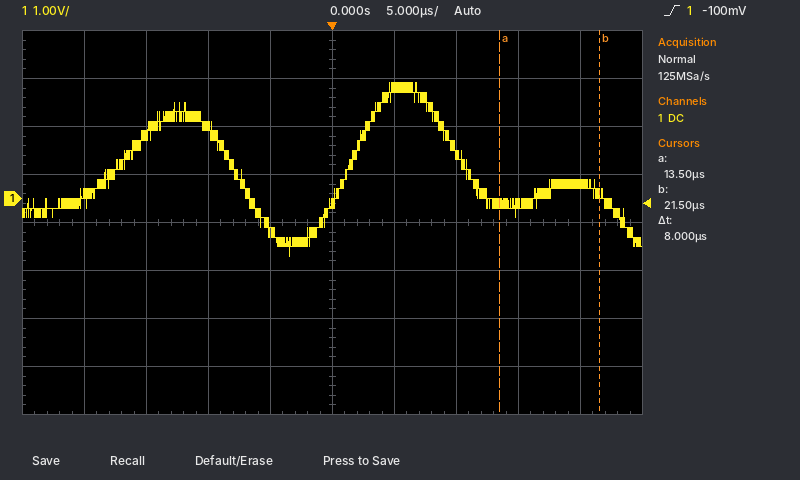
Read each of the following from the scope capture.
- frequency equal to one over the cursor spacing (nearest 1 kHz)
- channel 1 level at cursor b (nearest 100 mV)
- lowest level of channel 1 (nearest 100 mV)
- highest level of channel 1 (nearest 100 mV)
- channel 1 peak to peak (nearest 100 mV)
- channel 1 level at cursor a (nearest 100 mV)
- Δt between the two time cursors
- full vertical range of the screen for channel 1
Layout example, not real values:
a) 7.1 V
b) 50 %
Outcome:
a) 125 kHz
b) 100 mV
c) -1.2 V
d) 2.4 V
e) 3.6 V
f) -100 mV
g) 8 µs
h) 8 V
